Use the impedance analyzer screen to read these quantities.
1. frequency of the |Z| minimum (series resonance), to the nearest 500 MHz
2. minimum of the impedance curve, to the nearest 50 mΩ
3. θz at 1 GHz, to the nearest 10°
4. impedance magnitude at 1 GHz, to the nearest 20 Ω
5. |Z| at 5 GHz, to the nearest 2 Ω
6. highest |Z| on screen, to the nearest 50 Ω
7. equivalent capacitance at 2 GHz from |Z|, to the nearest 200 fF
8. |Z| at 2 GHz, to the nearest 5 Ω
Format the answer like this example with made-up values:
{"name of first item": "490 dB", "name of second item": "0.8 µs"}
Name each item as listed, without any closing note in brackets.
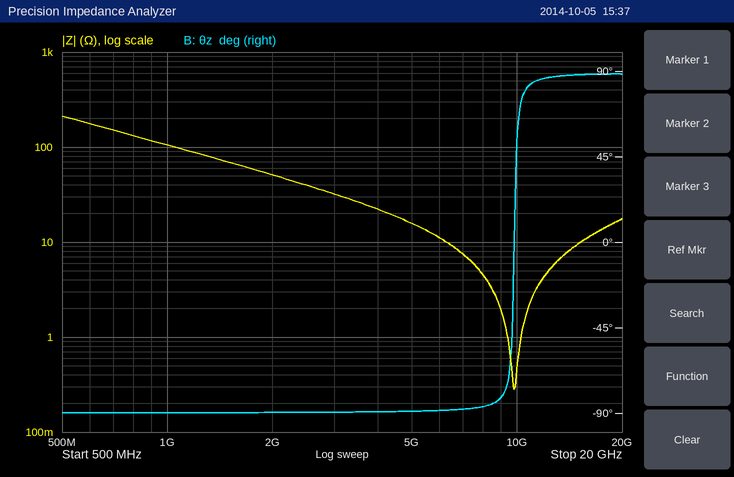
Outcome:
{"frequency of the |Z| minimum (series resonance), to the nearest 500 MHz": "10.0 GHz", "minimum of the impedance curve, to the nearest 50 mΩ": "300 mΩ", "θz at 1 GHz, to the nearest 10°": "-90°", "impedance magnitude at 1 GHz, to the nearest 20 Ω": "100 Ω", "|Z| at 5 GHz, to the nearest 2 Ω": "16 Ω", "highest |Z| on screen, to the nearest 50 Ω": "200 Ω", "equivalent capacitance at 2 GHz from |Z|, to the nearest 200 fF": "1.6 pF", "|Z| at 2 GHz, to the nearest 5 Ω": "50 Ω"}
